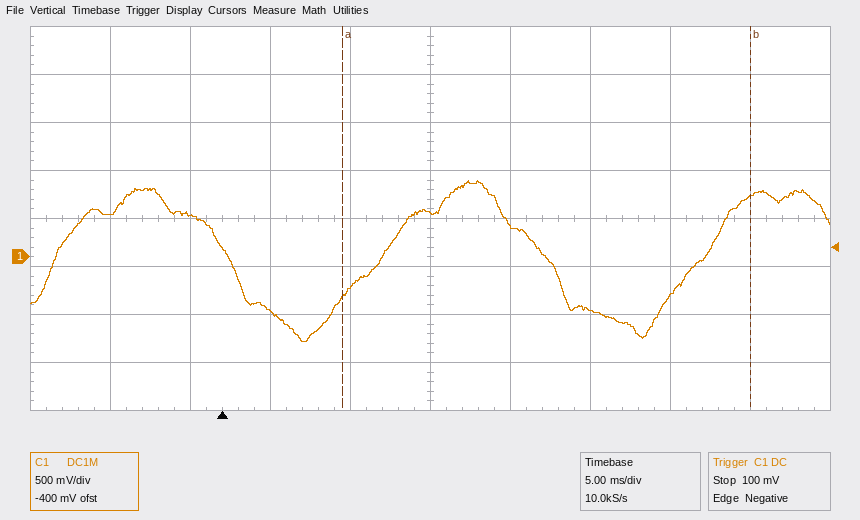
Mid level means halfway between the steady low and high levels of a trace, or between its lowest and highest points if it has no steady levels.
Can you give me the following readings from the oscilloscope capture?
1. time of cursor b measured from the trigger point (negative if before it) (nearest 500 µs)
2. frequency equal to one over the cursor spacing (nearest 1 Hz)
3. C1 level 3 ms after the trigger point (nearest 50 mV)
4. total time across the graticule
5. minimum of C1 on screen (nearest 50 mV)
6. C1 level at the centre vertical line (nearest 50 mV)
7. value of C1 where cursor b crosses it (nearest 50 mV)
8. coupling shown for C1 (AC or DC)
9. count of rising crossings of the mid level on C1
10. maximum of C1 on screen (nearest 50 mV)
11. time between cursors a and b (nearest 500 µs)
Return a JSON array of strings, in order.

["+33.0 ms", "39 Hz", "-550 mV", "50 ms", "-900 mV", "450 mV", "650 mV", "DC", "3", "800 mV", "25.5 ms"]
